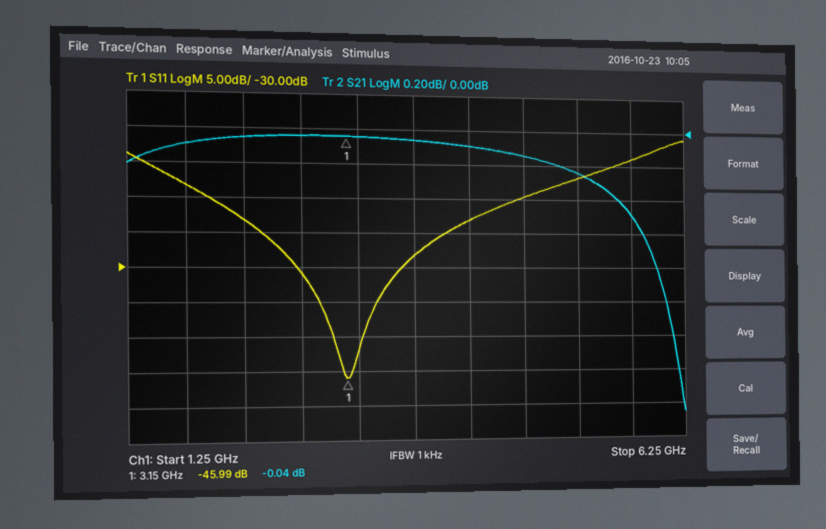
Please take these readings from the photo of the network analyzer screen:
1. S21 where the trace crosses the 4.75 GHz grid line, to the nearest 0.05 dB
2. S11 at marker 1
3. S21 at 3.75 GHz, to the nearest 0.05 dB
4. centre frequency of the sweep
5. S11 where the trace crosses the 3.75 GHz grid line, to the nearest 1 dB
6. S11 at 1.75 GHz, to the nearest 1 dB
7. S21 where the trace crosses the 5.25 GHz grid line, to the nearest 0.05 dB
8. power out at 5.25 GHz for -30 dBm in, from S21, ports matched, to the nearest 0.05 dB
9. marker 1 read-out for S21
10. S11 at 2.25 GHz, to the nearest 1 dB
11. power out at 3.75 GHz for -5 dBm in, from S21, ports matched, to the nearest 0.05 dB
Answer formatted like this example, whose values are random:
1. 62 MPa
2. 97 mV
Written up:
1. -0.15 dB
2. -45.99 dB
3. -0.05 dB
4. 3.75 GHz
5. -28 dB
6. -18 dB
7. -0.25 dB
8. -30.25 dBm
9. -0.04 dB
10. -23 dB
11. -5.05 dBm
